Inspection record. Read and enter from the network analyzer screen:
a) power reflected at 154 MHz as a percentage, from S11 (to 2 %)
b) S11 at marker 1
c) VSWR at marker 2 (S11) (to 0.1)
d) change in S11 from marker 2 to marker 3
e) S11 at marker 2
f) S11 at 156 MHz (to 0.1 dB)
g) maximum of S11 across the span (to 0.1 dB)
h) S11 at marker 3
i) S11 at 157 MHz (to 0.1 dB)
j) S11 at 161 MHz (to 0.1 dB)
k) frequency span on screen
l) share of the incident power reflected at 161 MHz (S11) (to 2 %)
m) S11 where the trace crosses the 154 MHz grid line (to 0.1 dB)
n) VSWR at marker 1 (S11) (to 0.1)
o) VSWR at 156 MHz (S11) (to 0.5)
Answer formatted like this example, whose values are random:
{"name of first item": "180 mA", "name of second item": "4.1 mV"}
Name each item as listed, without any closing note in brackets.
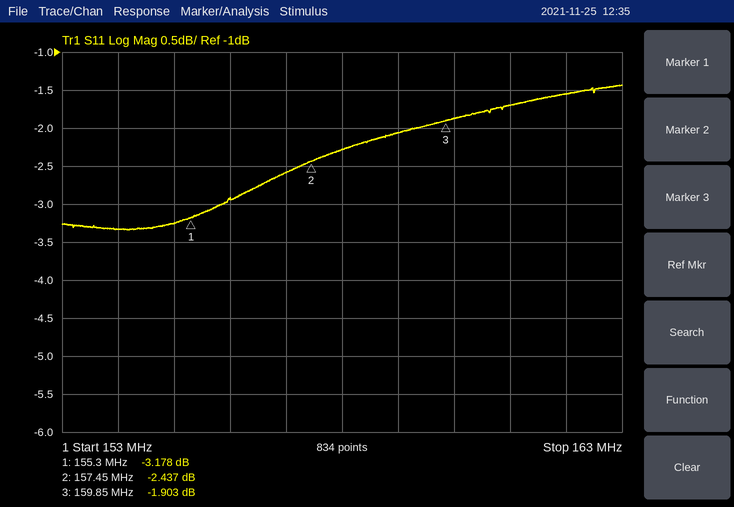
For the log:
{"power reflected at 154 MHz as a percentage, from S11": "46 %", "S11 at marker 1": "-3.178 dB", "VSWR at marker 2 (S11)": "7.2", "change in S11 from marker 2 to marker 3": "0.534 dB", "S11 at marker 2": "-2.437 dB", "S11 at 156 MHz": "-2.9 dB", "maximum of S11 across the span": "-1.4 dB", "S11 at marker 3": "-1.903 dB", "S11 at 157 MHz": "-2.6 dB", "S11 at 161 MHz": "-1.7 dB", "frequency span on screen": "10 MHz", "share of the incident power reflected at 161 MHz (S11)": "68 %", "S11 where the trace crosses the 154 MHz grid line": "-3.3 dB", "VSWR at marker 1 (S11)": "5.5", "VSWR at 156 MHz (S11)": "6.0"}
